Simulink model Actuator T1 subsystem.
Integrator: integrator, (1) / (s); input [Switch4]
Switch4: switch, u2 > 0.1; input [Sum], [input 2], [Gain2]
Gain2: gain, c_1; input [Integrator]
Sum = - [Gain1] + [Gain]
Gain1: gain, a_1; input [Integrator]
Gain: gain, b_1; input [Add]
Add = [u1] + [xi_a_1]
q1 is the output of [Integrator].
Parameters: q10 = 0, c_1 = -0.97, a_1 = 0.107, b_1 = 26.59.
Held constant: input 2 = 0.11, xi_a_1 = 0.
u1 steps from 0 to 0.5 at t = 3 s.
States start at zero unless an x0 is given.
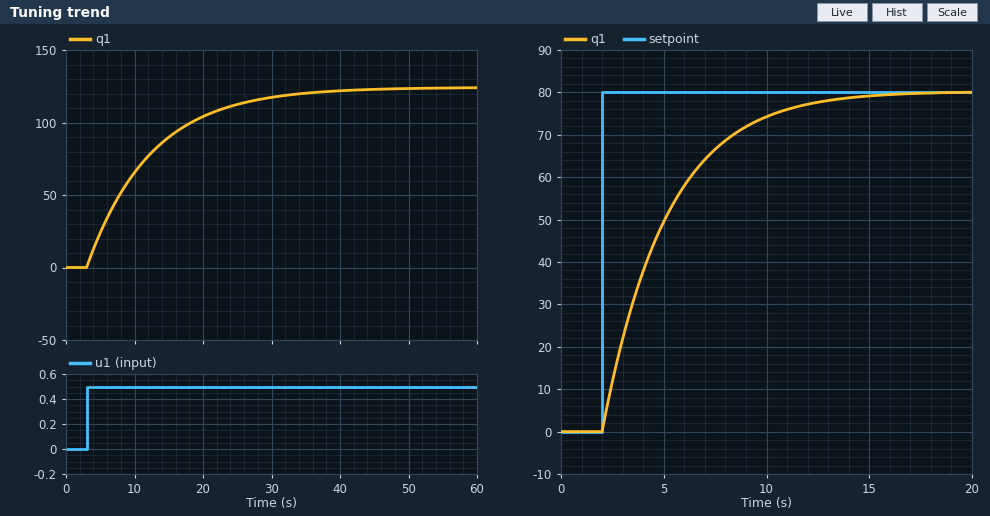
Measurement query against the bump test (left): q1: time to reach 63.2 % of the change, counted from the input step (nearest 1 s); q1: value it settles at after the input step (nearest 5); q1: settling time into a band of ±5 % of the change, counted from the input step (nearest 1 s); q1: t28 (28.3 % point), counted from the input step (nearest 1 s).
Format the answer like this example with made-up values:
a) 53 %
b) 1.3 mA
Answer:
a) 9 s
b) 125
c) 28 s
d) 3 s
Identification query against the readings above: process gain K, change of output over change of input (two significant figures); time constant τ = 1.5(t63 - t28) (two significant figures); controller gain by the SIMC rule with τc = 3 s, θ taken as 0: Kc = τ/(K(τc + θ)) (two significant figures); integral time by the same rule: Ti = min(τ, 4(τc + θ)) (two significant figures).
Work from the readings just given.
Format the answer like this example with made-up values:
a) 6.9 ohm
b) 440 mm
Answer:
a) 250
b) 9.0 s
c) 0.012
d) 9.0 s
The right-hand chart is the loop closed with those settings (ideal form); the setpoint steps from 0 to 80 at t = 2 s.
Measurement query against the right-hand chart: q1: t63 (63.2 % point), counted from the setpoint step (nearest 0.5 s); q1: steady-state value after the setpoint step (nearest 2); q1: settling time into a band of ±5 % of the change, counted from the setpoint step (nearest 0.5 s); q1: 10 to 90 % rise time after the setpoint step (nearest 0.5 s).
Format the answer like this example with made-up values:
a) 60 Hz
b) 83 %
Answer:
a) 3.0 s
b) 80
c) 9.0 s
d) 6.5 s
